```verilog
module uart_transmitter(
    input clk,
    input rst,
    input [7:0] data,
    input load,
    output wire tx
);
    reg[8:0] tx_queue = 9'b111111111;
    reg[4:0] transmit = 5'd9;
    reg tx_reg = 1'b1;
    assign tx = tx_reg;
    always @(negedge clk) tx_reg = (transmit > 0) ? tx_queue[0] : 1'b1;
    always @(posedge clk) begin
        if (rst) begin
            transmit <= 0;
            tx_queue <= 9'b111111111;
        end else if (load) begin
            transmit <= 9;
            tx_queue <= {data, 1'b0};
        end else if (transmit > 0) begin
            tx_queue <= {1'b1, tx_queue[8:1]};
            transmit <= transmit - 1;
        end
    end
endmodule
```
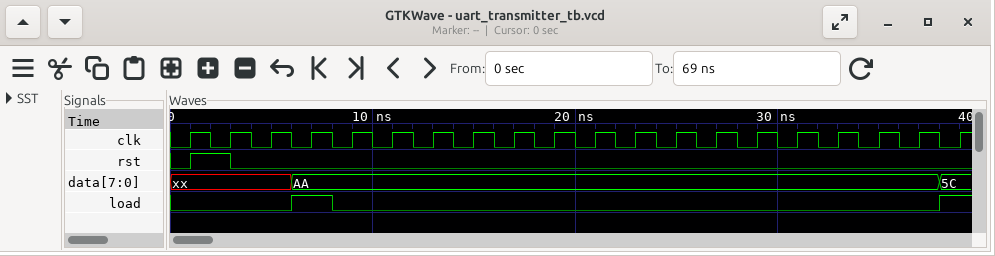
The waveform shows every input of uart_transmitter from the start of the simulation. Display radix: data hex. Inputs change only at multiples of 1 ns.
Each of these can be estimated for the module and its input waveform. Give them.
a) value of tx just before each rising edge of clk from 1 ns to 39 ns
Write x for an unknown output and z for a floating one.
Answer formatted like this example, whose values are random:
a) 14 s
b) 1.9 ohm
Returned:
a) 1 1 1 1 0 0 1 0 1 0 1 0 1 1 1 1 1 1 1 1
